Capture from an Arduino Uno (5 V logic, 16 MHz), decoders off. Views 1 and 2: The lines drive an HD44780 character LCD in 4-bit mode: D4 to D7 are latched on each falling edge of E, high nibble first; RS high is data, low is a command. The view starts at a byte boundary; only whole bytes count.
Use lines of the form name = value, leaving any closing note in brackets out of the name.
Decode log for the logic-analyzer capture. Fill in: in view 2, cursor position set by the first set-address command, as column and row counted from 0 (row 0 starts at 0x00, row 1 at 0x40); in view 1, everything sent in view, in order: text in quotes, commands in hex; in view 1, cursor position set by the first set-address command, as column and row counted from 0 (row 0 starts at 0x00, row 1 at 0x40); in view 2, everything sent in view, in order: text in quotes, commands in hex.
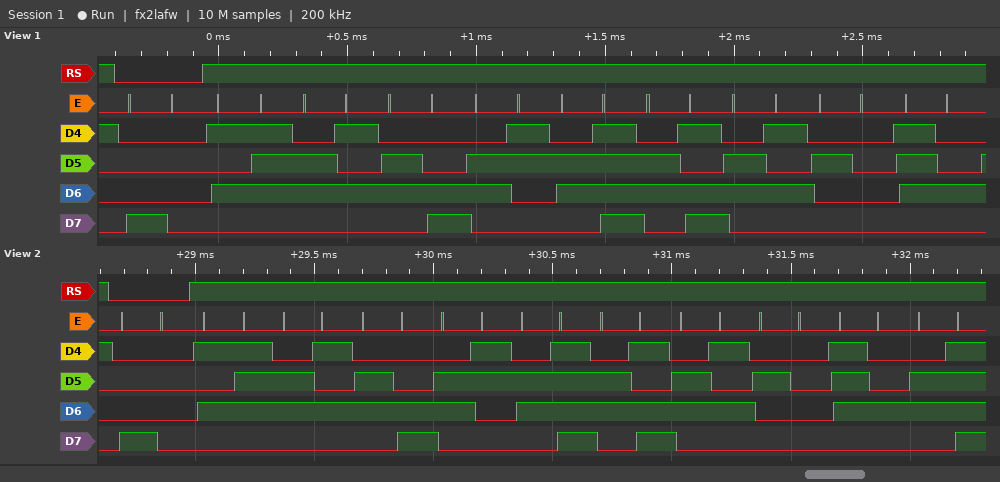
in view 2, cursor position set by the first set-address command, as column and row counted from 0 = column 0, row 0
in view 1, everything sent in view, in order: text in quotes, commands in hex = 0x80 "Welcome t"
in view 1, cursor position set by the first set-address command, as column and row counted from 0 = column 0, row 0
in view 2, everything sent in view, in order: text in quotes, commands in hex = 0x80 "Welcome to"
